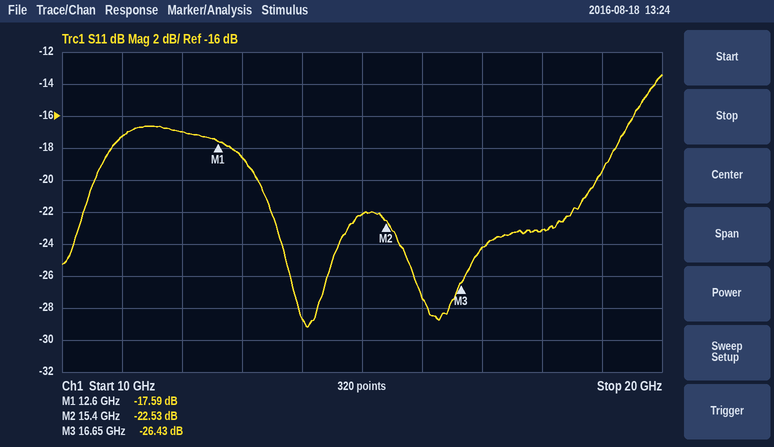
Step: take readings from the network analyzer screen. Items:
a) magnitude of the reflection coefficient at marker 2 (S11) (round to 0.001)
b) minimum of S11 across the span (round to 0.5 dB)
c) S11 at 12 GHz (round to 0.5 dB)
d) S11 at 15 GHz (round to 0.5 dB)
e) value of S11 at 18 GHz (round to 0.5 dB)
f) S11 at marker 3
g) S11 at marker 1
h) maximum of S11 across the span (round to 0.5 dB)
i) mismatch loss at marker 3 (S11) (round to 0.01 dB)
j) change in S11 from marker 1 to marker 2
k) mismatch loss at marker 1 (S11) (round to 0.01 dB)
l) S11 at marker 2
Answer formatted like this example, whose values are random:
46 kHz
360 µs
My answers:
0.075
-29.0 dB
-17.0 dB
-22.0 dB
-23.0 dB
-26.43 dB
-17.59 dB
-13.5 dB
0.01 dB
-4.94 dB
0.08 dB
-22.53 dB
